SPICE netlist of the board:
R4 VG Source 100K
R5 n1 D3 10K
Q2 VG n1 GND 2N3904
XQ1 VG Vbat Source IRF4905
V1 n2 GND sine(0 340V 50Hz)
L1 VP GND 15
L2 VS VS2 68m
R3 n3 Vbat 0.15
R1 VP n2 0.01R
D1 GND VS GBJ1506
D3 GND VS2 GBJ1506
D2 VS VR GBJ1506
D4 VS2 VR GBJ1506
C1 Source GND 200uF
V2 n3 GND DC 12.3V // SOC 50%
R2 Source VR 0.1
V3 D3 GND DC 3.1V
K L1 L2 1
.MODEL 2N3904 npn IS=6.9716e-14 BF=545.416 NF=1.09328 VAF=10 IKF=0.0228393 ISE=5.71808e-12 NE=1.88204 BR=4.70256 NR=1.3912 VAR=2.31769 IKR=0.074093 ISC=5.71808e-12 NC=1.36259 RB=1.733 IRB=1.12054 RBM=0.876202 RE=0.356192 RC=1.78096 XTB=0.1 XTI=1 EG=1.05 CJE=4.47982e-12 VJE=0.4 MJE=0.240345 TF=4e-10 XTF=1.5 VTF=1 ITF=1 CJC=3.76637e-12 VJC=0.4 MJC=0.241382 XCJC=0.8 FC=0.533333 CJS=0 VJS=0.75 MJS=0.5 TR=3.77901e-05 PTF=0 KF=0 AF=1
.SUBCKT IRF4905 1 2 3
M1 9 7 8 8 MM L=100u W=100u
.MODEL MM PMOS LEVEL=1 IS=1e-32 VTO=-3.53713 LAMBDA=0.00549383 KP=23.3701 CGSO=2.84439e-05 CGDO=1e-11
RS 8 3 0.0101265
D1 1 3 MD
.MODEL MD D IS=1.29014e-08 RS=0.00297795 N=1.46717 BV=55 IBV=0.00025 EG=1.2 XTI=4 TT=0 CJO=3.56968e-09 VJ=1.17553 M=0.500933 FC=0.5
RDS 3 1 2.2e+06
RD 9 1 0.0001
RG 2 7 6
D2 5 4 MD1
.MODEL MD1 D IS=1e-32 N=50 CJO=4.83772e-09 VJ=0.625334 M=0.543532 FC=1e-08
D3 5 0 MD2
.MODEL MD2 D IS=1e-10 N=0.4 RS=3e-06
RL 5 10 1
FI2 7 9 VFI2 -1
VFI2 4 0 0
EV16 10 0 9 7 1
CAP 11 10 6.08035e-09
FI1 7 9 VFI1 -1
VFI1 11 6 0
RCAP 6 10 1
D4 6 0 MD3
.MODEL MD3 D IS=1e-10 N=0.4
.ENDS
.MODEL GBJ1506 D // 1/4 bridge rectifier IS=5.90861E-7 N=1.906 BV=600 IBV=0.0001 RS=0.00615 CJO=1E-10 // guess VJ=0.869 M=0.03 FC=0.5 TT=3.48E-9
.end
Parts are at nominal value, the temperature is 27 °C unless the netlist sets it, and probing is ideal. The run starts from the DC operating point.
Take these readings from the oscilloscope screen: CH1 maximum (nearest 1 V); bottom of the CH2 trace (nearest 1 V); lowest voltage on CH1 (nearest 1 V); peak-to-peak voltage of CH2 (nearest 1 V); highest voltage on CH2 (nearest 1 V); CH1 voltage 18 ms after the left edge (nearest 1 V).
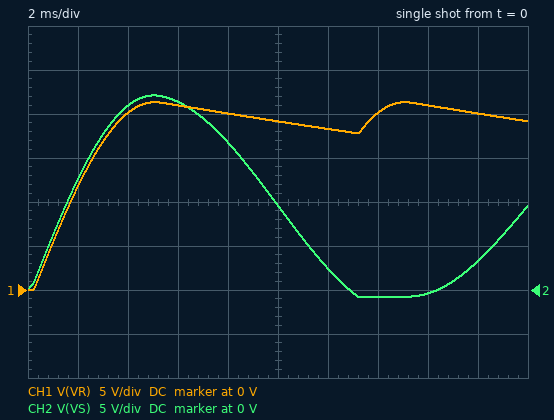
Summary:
21 V
-1 V
0 V
23 V
22 V
20 V
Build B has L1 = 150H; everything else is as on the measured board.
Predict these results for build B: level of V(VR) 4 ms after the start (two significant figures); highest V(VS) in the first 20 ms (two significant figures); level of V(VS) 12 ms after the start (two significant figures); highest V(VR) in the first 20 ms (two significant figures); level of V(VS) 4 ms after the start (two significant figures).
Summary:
5.3 V
6.5 V
760 mV
5.8 V
6.1 V
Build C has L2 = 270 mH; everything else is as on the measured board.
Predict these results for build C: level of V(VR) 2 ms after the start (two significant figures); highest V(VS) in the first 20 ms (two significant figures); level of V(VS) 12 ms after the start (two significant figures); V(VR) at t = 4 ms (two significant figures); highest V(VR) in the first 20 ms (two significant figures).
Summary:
25 V
45 V
5.8 V
42 V
44 V
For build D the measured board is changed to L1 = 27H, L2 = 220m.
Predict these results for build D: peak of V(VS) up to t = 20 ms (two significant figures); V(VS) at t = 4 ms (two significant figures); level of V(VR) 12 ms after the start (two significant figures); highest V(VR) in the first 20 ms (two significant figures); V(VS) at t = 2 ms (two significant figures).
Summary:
30 V
28 V
25 V
29 V
17 V
